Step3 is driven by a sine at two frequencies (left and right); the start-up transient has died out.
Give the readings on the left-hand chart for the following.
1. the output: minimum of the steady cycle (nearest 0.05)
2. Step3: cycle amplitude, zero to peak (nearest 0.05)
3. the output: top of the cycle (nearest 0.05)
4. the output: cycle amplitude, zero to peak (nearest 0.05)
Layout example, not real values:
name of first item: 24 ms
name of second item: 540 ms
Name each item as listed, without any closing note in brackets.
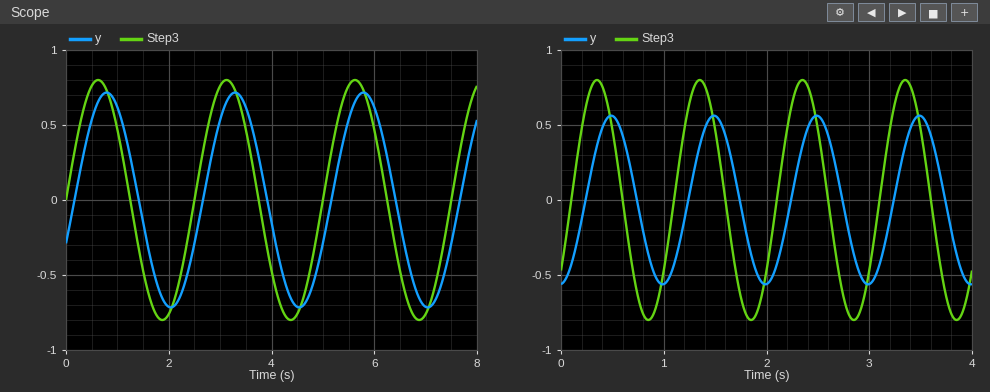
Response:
the output: minimum of the steady cycle: -0.70
Step3: cycle amplitude, zero to peak: 0.80
the output: top of the cycle: 0.70
the output: cycle amplitude, zero to peak: 0.70
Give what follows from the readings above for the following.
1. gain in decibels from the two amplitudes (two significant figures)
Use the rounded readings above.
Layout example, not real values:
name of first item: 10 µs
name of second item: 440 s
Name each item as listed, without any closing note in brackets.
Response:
gain in decibels from the two amplitudes: -1.2 dB
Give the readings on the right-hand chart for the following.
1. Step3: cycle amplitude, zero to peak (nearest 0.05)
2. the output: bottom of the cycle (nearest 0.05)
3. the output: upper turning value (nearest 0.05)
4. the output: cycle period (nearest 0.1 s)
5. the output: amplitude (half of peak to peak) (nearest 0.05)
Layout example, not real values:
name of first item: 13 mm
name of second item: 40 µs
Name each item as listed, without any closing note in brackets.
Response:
Step3: cycle amplitude, zero to peak: 0.80
the output: bottom of the cycle: -0.55
the output: upper turning value: 0.55
the output: cycle period: 1.0 s
the output: amplitude (half of peak to peak): 0.55
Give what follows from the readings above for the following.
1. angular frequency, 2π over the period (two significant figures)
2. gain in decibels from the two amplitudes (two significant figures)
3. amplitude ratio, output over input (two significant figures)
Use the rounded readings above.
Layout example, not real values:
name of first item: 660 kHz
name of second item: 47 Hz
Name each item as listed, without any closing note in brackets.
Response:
angular frequency, 2π over the period: 6.3 rad/s
gain in decibels from the two amplitudes: -3.3 dB
amplitude ratio, output over input: 0.69
